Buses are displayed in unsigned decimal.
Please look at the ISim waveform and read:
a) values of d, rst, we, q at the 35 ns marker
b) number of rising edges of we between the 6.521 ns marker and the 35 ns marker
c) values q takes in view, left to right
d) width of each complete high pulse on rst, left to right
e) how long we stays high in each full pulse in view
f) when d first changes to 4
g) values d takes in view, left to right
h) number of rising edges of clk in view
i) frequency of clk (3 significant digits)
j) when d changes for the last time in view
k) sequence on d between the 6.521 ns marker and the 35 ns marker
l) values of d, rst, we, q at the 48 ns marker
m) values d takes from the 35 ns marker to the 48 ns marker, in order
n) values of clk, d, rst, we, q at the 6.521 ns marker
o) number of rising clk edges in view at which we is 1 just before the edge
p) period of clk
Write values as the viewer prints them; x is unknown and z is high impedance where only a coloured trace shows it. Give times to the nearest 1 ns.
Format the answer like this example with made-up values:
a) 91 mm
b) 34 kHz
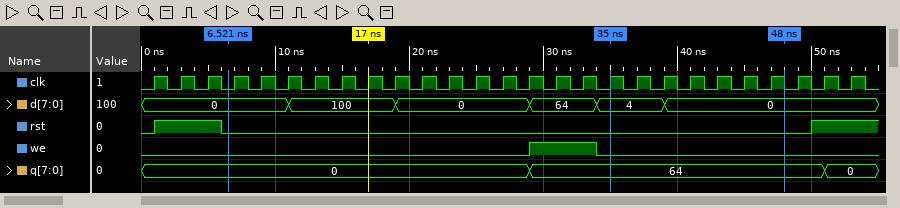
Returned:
a) d=4, rst=0, we=0, q=64
b) 1
c) 0, 64, 0
d) 5 ns
e) 5 ns
f) 34 ns
g) 0, 100, 0, 64, 4, 0
h) 27
i) 500 MHz
j) 39 ns
k) 0, 100, 0, 64, 4
l) d=0, rst=0, we=0, q=64
m) 4, 0
n) clk=0, d=0, rst=0, we=0, q=0
o) 2
p) 2 ns
